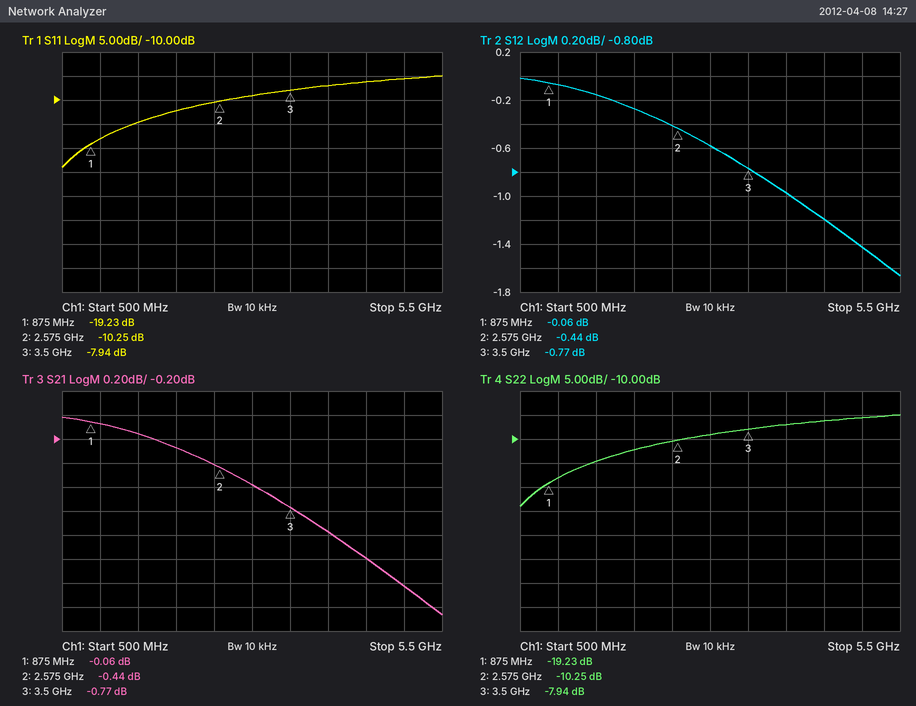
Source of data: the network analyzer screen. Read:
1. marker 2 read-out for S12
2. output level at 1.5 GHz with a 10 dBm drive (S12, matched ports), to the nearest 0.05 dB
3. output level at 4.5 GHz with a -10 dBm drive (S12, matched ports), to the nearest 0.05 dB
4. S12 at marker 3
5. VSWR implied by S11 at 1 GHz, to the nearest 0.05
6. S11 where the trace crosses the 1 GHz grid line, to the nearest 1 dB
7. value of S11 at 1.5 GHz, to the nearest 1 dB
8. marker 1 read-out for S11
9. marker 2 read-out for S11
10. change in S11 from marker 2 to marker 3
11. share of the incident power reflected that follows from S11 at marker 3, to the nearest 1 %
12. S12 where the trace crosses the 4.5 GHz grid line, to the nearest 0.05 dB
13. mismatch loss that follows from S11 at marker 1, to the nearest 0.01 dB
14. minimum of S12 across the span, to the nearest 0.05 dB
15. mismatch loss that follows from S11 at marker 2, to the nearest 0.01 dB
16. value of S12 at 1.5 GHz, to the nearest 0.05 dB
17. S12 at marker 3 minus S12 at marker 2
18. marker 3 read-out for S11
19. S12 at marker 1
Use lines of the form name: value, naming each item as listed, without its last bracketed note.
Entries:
marker 2 read-out for S12: -0.44 dB
output level at 1.5 GHz with a 10 dBm drive (S12, matched ports), to the nearest 0.05 dB: 9.85 dBm
output level at 4.5 GHz with a -10 dBm drive (S12, matched ports), to the nearest 0.05 dB: -11.20 dBm
S12 at marker 3: -0.77 dB
VSWR implied by S11 at 1 GHz, to the nearest 0.05: 1.30
S11 where the trace crosses the 1 GHz grid line, to the nearest 1 dB: -18 dB
value of S11 at 1.5 GHz, to the nearest 1 dB: -15 dB
marker 1 read-out for S11: -19.23 dB
marker 2 read-out for S11: -10.25 dB
change in S11 from marker 2 to marker 3: 2.31 dB
share of the incident power reflected that follows from S11 at marker 3, to the nearest 1 %: 16 %
S12 where the trace crosses the 4.5 GHz grid line, to the nearest 0.05 dB: -1.20 dB
mismatch loss that follows from S11 at marker 1, to the nearest 0.01 dB: 0.05 dB
minimum of S12 across the span, to the nearest 0.05 dB: -1.65 dB
mismatch loss that follows from S11 at marker 2, to the nearest 0.01 dB: 0.43 dB
value of S12 at 1.5 GHz, to the nearest 0.05 dB: -0.15 dB
S12 at marker 3 minus S12 at marker 2: -0.33 dB
marker 3 read-out for S11: -7.94 dB
S12 at marker 1: -0.06 dB
